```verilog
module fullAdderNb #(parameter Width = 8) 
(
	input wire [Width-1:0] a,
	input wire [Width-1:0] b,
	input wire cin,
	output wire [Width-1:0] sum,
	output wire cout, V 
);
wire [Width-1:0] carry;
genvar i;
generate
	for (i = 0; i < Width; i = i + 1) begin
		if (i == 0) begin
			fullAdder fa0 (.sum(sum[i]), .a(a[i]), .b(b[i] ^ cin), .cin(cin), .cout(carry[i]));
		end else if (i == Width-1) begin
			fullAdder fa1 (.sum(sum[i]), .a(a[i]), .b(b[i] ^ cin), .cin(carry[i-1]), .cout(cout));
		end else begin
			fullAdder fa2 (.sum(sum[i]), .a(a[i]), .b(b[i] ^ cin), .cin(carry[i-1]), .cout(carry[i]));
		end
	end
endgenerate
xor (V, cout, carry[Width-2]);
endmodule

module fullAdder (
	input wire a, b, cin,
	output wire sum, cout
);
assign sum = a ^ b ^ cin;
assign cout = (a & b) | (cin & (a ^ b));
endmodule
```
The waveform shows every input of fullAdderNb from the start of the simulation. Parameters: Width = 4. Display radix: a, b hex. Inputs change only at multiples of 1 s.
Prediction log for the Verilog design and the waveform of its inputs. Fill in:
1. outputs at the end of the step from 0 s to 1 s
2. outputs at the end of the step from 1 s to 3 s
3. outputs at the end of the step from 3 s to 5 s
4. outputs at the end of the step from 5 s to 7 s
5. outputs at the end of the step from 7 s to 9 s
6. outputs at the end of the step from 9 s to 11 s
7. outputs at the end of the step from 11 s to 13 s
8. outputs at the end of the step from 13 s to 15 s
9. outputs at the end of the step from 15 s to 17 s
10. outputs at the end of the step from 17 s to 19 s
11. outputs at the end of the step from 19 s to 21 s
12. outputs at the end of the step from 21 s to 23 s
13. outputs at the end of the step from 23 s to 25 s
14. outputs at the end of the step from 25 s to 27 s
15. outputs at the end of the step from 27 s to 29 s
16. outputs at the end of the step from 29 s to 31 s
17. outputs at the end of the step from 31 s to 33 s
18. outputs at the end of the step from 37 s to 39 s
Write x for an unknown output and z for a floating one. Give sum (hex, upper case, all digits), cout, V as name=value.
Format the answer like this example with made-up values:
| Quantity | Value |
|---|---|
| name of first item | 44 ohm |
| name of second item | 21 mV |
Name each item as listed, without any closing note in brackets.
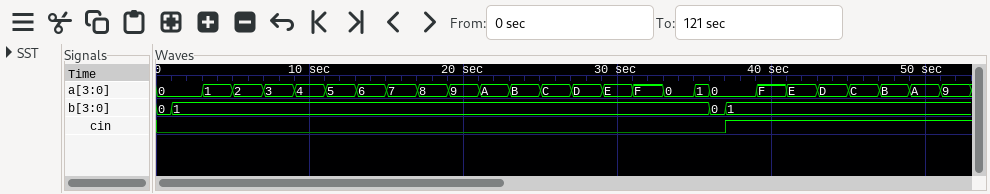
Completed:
| Quantity | Value |
|---|---|
| outputs at the end of the step from 0 s to 1 s | sum=0, cout=0, V=0 |
| outputs at the end of the step from 1 s to 3 s | sum=1, cout=0, V=0 |
| outputs at the end of the step from 3 s to 5 s | sum=2, cout=0, V=0 |
| outputs at the end of the step from 5 s to 7 s | sum=3, cout=0, V=0 |
| outputs at the end of the step from 7 s to 9 s | sum=4, cout=0, V=0 |
| outputs at the end of the step from 9 s to 11 s | sum=5, cout=0, V=0 |
| outputs at the end of the step from 11 s to 13 s | sum=6, cout=0, V=0 |
| outputs at the end of the step from 13 s to 15 s | sum=7, cout=0, V=0 |
| outputs at the end of the step from 15 s to 17 s | sum=8, cout=0, V=1 |
| outputs at the end of the step from 17 s to 19 s | sum=9, cout=0, V=0 |
| outputs at the end of the step from 19 s to 21 s | sum=A, cout=0, V=0 |
| outputs at the end of the step from 21 s to 23 s | sum=B, cout=0, V=0 |
| outputs at the end of the step from 23 s to 25 s | sum=C, cout=0, V=0 |
| outputs at the end of the step from 25 s to 27 s | sum=D, cout=0, V=0 |
| outputs at the end of the step from 27 s to 29 s | sum=E, cout=0, V=0 |
| outputs at the end of the step from 29 s to 31 s | sum=F, cout=0, V=0 |
| outputs at the end of the step from 31 s to 33 s | sum=0, cout=1, V=0 |
| outputs at the end of the step from 37 s to 39 s | sum=F, cout=0, V=0 |
